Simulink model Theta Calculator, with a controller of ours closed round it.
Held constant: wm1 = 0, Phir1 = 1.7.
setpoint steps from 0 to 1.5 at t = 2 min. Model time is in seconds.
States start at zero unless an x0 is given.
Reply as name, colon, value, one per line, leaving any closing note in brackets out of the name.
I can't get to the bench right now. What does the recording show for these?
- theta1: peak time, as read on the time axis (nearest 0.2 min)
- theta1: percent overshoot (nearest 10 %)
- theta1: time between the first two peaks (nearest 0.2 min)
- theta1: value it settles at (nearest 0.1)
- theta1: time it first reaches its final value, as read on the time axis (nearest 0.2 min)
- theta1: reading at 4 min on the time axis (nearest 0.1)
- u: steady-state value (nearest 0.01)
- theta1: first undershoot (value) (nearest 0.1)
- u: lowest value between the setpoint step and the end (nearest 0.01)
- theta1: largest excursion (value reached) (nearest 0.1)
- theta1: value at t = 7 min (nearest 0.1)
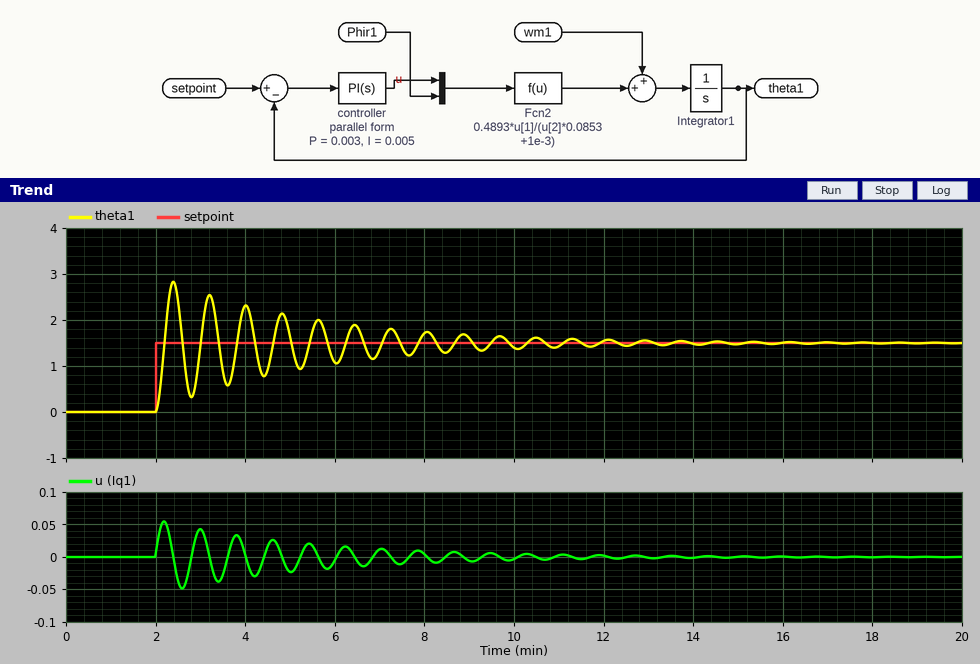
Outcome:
theta1: peak time, as read on the time axis: 2.4 min
theta1: percent overshoot: 90 %
theta1: time between the first two peaks: 0.8 min
theta1: value it settles at: 1.5
theta1: time it first reaches its final value, as read on the time axis: 2.2 min
theta1: reading at 4 min on the time axis: 2.3
u: steady-state value: 0.00
theta1: first undershoot (value): 0.3
u: lowest value between the setpoint step and the end: -0.05
theta1: largest excursion (value reached): 2.8
theta1: value at t = 7 min: 1.4
